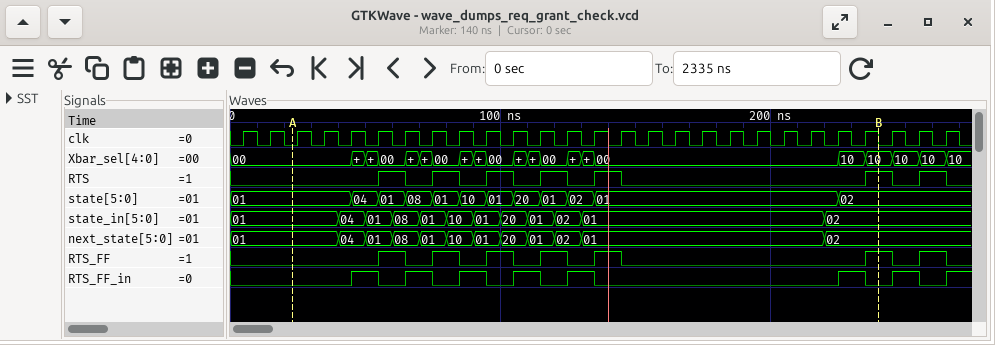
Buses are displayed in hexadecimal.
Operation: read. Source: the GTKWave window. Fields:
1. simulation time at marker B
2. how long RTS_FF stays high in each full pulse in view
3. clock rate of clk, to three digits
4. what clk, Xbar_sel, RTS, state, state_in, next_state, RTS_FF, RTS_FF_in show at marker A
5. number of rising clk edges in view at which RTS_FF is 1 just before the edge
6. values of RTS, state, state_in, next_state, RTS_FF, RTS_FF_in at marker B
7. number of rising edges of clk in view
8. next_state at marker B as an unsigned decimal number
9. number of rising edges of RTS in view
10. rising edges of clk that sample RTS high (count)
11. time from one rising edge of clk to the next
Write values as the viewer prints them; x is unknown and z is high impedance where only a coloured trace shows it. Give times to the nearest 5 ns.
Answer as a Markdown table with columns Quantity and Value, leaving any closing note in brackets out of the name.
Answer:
| Quantity | Value |
|---|---|
| simulation time at marker B | 240 ns |
| how long RTS_FF stays high in each full pulse in view | 10 ns, 10 ns, 10 ns, 10 ns, 10 ns, 10 ns, 10 ns |
| clock rate of clk, to three digits | 100 MHz |
| what clk, Xbar_sel, RTS, state, state_in, next_state, RTS_FF, RTS_FF_in show at marker A | clk=0, Xbar_sel=00, RTS=0, state=01, state_in=01, next_state=01, RTS_FF=0, RTS_FF_in=0 |
| number of rising clk edges in view at which RTS_FF is 1 just before the edge | 7 |
| values of RTS, state, state_in, next_state, RTS_FF, RTS_FF_in at marker B | RTS=1, state=02, state_in=02, next_state=02, RTS_FF=1, RTS_FF_in=0 |
| number of rising edges of clk in view | 27 |
| next_state at marker B as an unsigned decimal number | 2 |
| number of rising edges of RTS in view | 7 |
| rising edges of clk that sample RTS high | 7 |
| time from one rising edge of clk to the next | 10 ns |
